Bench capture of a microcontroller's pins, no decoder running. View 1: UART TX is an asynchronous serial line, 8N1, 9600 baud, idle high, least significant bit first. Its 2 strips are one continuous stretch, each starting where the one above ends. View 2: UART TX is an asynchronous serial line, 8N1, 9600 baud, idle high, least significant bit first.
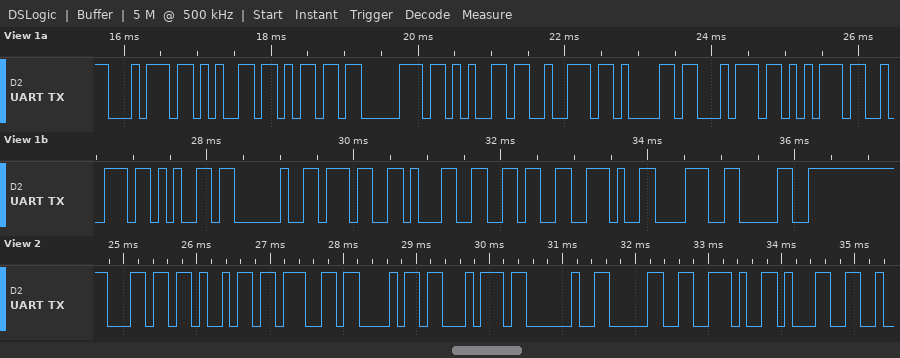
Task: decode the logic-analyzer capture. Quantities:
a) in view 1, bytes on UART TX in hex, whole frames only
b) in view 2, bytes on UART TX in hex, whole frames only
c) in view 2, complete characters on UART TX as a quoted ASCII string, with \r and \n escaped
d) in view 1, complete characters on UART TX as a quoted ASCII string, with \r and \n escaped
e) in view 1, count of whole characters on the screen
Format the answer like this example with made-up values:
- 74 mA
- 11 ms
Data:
- 74 65 6D 70 65 72 61 74 75 72 65 20 37 31 36 2E 38 30
- 0x6C 0x69 0x67 0x68 0x74 0x20 0x30 0x2E 0x31
- "light 0.1"
- "temperature 716.80"
- 18
